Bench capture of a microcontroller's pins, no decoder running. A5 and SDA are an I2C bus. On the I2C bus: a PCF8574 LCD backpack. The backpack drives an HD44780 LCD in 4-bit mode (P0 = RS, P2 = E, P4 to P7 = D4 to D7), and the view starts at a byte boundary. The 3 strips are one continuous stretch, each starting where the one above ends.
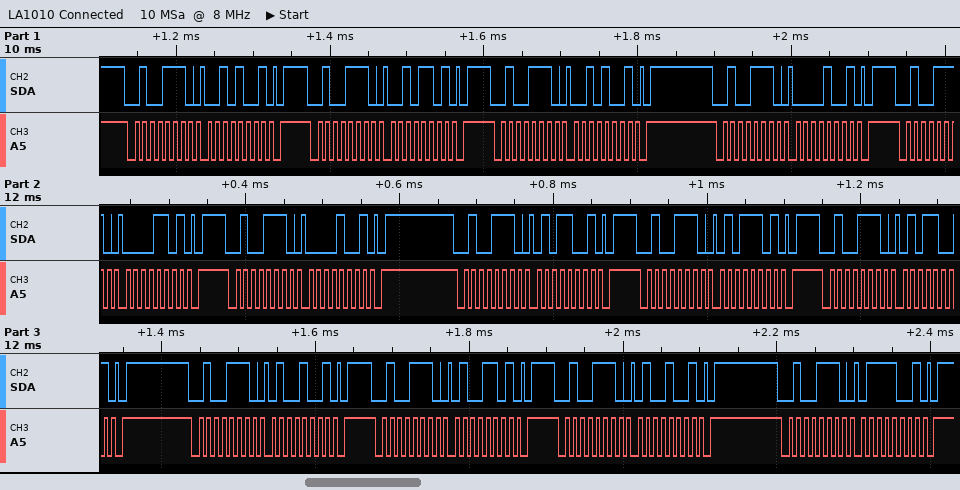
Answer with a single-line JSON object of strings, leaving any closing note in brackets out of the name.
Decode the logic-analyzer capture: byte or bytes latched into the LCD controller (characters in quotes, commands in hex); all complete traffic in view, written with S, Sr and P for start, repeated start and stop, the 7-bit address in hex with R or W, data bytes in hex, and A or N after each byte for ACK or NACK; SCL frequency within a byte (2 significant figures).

{"byte or bytes latched into the LCD controller": "' ' 'T'", "all complete traffic in view, written with S, Sr and P for start, repeated start and stop, the 7-bit address in hex with R or W, data bytes in hex, and A or N after each byte for ACK or NACK": "S 27W A 29 A P S 27W A 2D A P S 27W A 29 A P S 27W A 09 A P S 27W A 0D A P S 27W A 09 A P S 27W A 59 A P S 27W A 5D A P S 27W A 59 A P S 27W A 49 A P S 27W A 4D A P S 27W A 49 A P S 27W A 79 A P", "SCL frequency within a byte": "100 kHz"}
